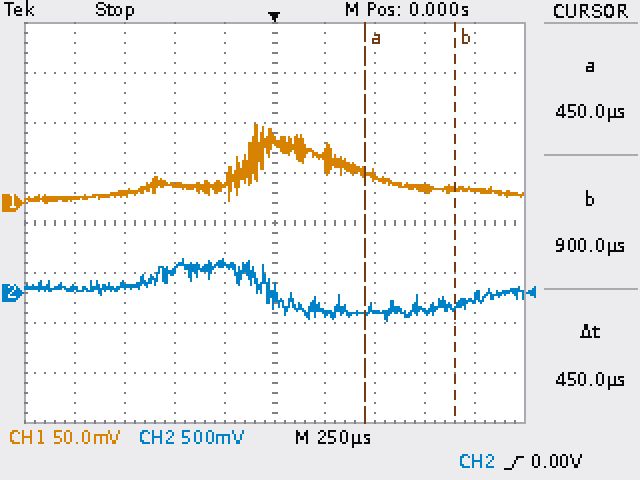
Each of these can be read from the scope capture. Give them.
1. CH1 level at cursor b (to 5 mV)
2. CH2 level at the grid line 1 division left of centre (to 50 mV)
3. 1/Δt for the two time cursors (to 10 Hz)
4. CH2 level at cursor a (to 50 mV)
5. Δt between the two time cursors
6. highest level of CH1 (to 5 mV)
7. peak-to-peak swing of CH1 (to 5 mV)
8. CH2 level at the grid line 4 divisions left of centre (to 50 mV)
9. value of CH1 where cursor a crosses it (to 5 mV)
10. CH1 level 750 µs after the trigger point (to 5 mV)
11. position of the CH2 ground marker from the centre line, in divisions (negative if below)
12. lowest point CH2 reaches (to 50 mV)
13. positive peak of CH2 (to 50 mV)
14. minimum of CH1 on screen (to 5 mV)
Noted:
15 mV
300 mV
2.22 kHz
-150 mV
450 µs
80 mV
80 mV
50 mV
30 mV
15 mV
-1.4 div
-300 mV
350 mV
0 mV
